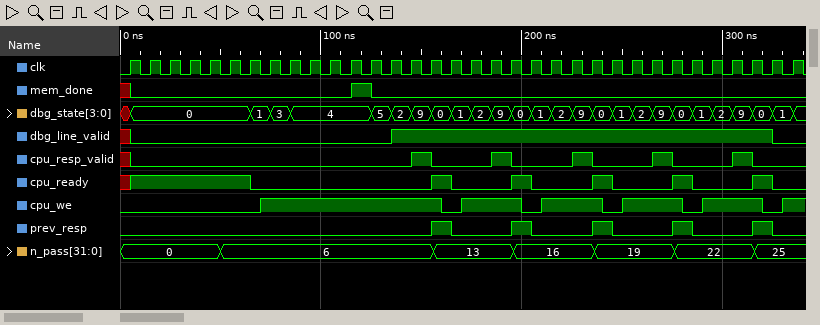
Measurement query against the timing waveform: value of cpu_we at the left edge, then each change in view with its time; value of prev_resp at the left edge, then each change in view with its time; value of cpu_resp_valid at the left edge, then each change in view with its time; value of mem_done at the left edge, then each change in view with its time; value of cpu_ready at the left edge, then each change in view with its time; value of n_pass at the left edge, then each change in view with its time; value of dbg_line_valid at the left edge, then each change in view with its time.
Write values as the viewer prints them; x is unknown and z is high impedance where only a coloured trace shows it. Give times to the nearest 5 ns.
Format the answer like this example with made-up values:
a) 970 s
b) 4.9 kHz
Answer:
a) 0, 1 at 70 ns, 0 at 160 ns, 1 at 170 ns, 0 at 200 ns, 1 at 210 ns, 0 at 240 ns, 1 at 250 ns, 0 at 280 ns, 1 at 290 ns, 0 at 320 ns, 1 at 330 ns
b) 0, 1 at 155 ns, 0 at 165 ns, 1 at 195 ns, 0 at 205 ns, 1 at 235 ns, 0 at 245 ns, 1 at 275 ns, 0 at 285 ns, 1 at 315 ns, 0 at 325 ns
c) x, 0 at 5 ns, 1 at 145 ns, 0 at 155 ns, 1 at 185 ns, 0 at 195 ns, 1 at 225 ns, 0 at 235 ns, 1 at 265 ns, 0 at 275 ns, 1 at 305 ns, 0 at 315 ns
d) x, 0 at 5 ns, 1 at 115 ns, 0 at 125 ns
e) x, 1 at 5 ns, 0 at 65 ns, 1 at 155 ns, 0 at 165 ns, 1 at 195 ns, 0 at 205 ns, 1 at 235 ns, 0 at 245 ns, 1 at 275 ns, 0 at 285 ns, 1 at 315 ns, 0 at 325 ns
f) 0, 6 at 50 ns, 13 at 155 ns, 16 at 195 ns, 19 at 235 ns, 22 at 275 ns, 25 at 315 ns
g) x, 0 at 5 ns, 1 at 135 ns, 0 at 325 ns
